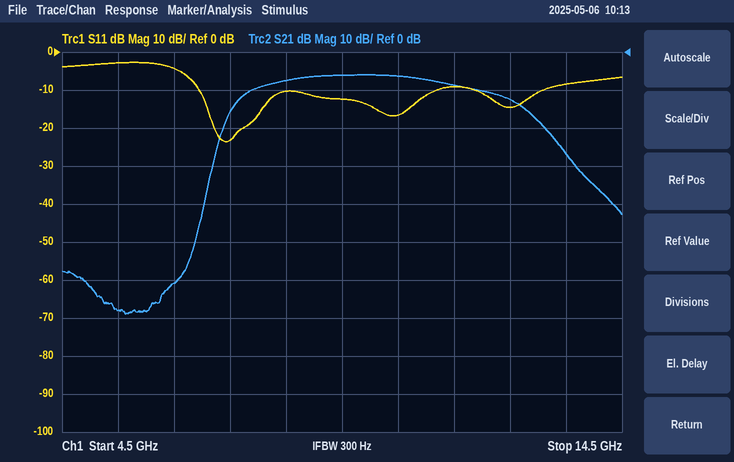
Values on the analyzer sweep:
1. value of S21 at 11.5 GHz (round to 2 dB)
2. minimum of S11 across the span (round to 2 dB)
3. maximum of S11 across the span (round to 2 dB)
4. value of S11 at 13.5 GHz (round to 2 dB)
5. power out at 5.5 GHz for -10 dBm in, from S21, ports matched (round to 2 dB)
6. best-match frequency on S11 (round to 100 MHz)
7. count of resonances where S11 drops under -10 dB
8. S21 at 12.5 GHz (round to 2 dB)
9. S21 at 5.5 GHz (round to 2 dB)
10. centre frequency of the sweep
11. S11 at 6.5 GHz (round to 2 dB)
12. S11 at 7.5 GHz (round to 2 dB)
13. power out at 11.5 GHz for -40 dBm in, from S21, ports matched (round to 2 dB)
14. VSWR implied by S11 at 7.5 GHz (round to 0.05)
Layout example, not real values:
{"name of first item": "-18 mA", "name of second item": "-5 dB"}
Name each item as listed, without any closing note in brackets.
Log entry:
{"value of S21 at 11.5 GHz": "-8 dB", "minimum of S11 across the span": "-24 dB", "maximum of S11 across the span": "-2 dB", "value of S11 at 13.5 GHz": "-8 dB", "power out at 5.5 GHz for -10 dBm in, from S21, ports matched": "-78 dBm", "best-match frequency on S11": "7.4 GHz", "count of resonances where S11 drops under -10 dB": "3", "S21 at 12.5 GHz": "-12 dB", "S21 at 5.5 GHz": "-68 dB", "centre frequency of the sweep": "9.5 GHz", "S11 at 6.5 GHz": "-4 dB", "S11 at 7.5 GHz": "-24 dB", "power out at 11.5 GHz for -40 dBm in, from S21, ports matched": "-48 dBm", "VSWR implied by S11 at 7.5 GHz": "1.15"}
